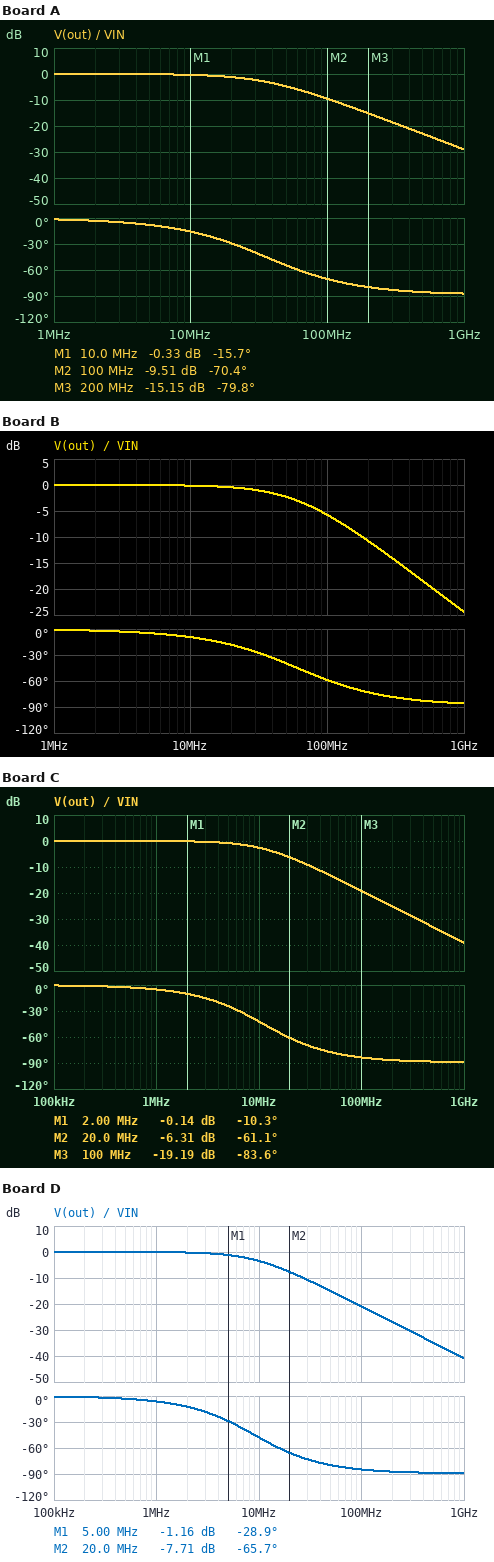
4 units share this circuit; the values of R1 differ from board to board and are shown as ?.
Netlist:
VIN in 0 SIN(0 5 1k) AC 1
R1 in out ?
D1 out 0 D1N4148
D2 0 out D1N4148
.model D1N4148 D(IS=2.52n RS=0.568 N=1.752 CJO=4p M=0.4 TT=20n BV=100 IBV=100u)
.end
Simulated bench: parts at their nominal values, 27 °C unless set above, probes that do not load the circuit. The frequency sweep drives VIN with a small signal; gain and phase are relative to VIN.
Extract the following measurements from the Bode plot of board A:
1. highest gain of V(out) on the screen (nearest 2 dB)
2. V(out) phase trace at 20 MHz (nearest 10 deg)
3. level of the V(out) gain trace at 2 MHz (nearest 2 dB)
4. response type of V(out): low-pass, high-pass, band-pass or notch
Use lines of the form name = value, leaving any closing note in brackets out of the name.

highest gain of V(out) on the screen = 0 dB
V(out) phase trace at 20 MHz = -30 deg
level of the V(out) gain trace at 2 MHz = 0 dB
response type of V(out): low-pass, high-pass, band-pass or notch = low-pass
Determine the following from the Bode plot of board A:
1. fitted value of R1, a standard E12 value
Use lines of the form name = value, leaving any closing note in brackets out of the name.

fitted value of R1, a standard E12 value = 560 Ω
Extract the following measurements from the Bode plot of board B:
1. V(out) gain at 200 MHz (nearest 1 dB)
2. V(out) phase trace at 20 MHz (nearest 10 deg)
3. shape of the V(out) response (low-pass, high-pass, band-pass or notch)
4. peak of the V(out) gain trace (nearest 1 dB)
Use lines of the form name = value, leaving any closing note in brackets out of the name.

V(out) gain at 200 MHz = -11 dB
V(out) phase trace at 20 MHz = -20 deg
shape of the V(out) response = low-pass
peak of the V(out) gain trace = 0 dB
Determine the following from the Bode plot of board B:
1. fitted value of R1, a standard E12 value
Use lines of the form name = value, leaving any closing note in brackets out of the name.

fitted value of R1, a standard E12 value = 330 Ω
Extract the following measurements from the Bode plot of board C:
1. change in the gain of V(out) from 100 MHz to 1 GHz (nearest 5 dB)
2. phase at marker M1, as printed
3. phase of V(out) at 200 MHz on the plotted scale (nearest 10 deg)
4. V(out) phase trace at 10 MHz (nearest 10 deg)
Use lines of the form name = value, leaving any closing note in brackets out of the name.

change in the gain of V(out) from 100 MHz to 1 GHz = -20 dB
phase at marker M1, as printed = -10.3 deg
phase of V(out) at 200 MHz on the plotted scale = -90 deg
V(out) phase trace at 10 MHz = -40 deg
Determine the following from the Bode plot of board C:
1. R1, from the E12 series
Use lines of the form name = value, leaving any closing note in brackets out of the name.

R1, from the E12 series = 1.8 kΩ
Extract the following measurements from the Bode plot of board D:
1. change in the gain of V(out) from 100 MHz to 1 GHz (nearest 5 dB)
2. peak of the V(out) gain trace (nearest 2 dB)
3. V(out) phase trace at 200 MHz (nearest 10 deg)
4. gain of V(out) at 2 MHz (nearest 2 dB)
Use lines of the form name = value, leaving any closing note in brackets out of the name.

change in the gain of V(out) from 100 MHz to 1 GHz = -20 dB
peak of the V(out) gain trace = 0 dB
V(out) phase trace at 200 MHz = -90 deg
gain of V(out) at 2 MHz = 0 dB
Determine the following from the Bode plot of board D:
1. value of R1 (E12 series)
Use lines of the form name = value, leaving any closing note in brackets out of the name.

value of R1 = 2.2 kΩ
